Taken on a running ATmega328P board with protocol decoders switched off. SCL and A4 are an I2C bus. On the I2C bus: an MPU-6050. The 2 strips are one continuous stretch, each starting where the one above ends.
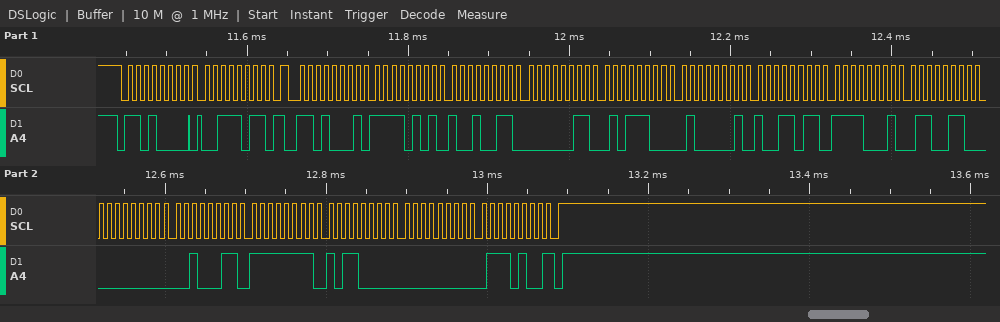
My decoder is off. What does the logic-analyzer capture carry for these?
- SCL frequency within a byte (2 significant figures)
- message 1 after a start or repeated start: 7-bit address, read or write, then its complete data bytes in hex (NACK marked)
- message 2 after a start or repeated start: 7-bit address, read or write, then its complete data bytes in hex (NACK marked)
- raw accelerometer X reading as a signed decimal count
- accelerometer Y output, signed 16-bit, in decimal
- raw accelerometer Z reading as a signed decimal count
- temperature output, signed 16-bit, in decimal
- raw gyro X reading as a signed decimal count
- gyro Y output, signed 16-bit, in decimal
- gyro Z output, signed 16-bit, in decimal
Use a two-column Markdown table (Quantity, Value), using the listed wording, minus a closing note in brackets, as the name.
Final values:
| Quantity | Value |
|---|---|
| SCL frequency within a byte | 100 kHz |
| message 1 after a start or repeated start: 7-bit address, read or write, then its complete data bytes in hex | 0x68 write: 3B |
| message 2 after a start or repeated start: 7-bit address, read or write, then its complete data bytes in hex | 0x68 read: F5 93 03 5C 41 9B F1 66 00 23 FF B0 00 74 NACK |
| raw accelerometer X reading as a signed decimal count | -2669 |
| accelerometer Y output, signed 16-bit, in decimal | 860 |
| raw accelerometer Z reading as a signed decimal count | 16795 |
| temperature output, signed 16-bit, in decimal | -3738 |
| raw gyro X reading as a signed decimal count | 35 |
| gyro Y output, signed 16-bit, in decimal | -80 |
| gyro Z output, signed 16-bit, in decimal | 116 |
